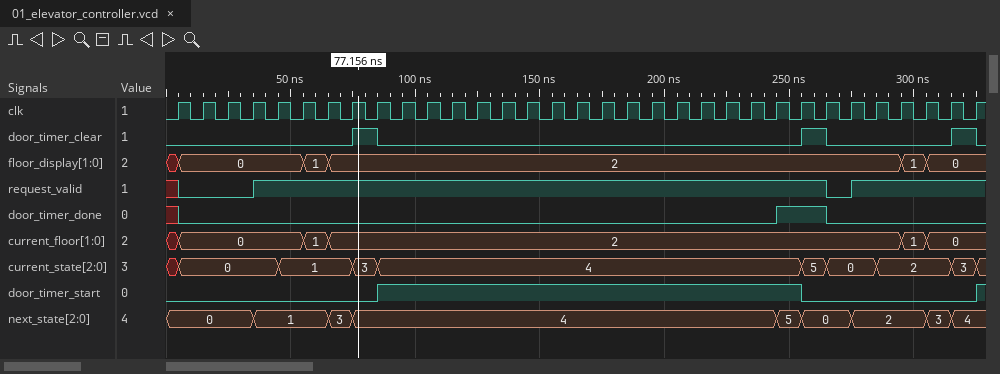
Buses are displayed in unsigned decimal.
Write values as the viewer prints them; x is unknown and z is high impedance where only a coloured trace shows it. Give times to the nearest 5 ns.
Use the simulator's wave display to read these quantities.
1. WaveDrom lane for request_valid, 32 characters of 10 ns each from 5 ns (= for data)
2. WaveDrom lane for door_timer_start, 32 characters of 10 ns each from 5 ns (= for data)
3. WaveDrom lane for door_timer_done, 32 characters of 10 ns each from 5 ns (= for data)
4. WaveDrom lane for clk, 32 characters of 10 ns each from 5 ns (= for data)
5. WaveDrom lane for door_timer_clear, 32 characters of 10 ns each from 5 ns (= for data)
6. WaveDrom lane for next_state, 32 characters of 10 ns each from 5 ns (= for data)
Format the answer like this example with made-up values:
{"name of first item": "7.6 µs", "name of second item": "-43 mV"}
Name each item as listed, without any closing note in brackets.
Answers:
{"WaveDrom lane for request_valid, 32 characters of 10 ns each from 5 ns": "{name: 'request_valid', wave: '0..1......................01....'}", "WaveDrom lane for door_timer_start, 32 characters of 10 ns each from 5 ns": "{name: 'door_timer_start', wave: '0.......1................0......'}", "WaveDrom lane for door_timer_done, 32 characters of 10 ns each from 5 ns": "{name: 'door_timer_done', wave: '0.......................1.0.....'}", "WaveDrom lane for clk, 32 characters of 10 ns each from 5 ns": "{name: 'clk', wave: 'p...............................'}", "WaveDrom lane for door_timer_clear, 32 characters of 10 ns each from 5 ns": "{name: 'door_timer_clear', wave: '0......10................10....1'}", "WaveDrom lane for next_state, 32 characters of 10 ns each from 5 ns": "{name: 'next_state', wave: '=..=..==................==.=..==', data: '0 1 3 4 5 0 2 3 4'}"}
